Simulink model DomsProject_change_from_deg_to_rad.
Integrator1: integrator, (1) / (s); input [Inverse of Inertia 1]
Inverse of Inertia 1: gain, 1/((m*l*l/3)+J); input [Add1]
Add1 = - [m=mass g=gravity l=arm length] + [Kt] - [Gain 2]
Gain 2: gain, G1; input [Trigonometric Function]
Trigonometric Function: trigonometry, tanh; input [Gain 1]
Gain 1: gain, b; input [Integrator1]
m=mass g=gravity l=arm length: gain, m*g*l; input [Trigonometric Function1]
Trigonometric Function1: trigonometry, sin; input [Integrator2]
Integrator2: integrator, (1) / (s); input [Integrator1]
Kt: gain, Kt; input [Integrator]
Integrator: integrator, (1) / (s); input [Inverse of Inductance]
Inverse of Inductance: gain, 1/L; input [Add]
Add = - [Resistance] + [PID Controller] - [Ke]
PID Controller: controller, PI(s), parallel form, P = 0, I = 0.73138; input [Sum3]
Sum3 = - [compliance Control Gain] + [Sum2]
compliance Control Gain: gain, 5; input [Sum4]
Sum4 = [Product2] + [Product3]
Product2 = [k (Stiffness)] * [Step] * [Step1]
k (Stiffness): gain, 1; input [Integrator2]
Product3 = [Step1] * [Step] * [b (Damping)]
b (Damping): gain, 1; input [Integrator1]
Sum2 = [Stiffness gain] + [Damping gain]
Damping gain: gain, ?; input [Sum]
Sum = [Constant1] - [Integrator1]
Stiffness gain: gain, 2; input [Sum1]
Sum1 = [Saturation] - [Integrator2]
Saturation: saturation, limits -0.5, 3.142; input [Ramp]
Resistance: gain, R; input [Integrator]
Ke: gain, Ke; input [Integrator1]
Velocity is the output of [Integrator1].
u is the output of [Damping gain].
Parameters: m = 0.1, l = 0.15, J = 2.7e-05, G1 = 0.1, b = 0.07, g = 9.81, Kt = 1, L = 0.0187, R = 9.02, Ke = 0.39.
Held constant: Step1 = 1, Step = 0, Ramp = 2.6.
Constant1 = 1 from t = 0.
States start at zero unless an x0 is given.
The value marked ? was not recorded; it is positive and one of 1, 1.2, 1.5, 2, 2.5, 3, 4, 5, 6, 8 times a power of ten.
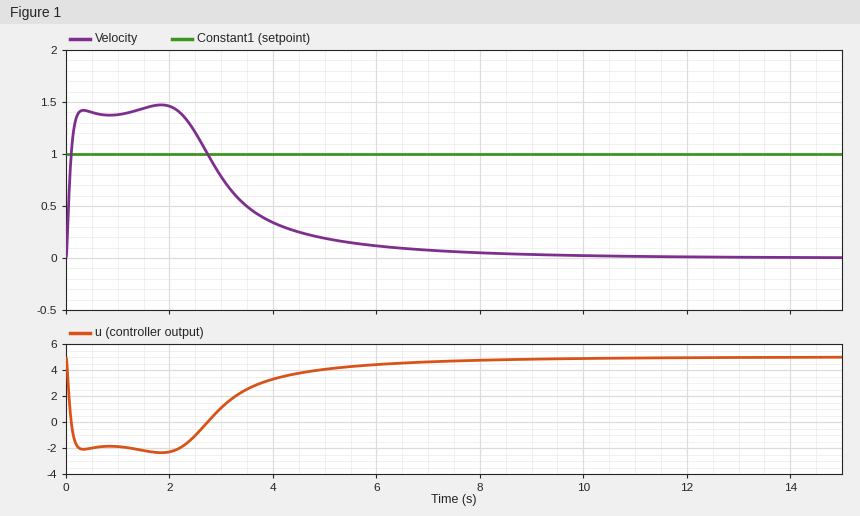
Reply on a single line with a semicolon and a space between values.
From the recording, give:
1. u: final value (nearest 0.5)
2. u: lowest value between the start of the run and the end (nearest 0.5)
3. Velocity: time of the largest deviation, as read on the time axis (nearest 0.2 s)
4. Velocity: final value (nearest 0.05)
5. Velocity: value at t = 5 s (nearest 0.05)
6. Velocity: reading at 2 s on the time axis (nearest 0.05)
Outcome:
5.0; -2.5; 1.8 s; 0.00; 0.20; 1.45
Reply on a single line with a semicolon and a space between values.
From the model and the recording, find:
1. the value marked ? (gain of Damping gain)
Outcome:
5
